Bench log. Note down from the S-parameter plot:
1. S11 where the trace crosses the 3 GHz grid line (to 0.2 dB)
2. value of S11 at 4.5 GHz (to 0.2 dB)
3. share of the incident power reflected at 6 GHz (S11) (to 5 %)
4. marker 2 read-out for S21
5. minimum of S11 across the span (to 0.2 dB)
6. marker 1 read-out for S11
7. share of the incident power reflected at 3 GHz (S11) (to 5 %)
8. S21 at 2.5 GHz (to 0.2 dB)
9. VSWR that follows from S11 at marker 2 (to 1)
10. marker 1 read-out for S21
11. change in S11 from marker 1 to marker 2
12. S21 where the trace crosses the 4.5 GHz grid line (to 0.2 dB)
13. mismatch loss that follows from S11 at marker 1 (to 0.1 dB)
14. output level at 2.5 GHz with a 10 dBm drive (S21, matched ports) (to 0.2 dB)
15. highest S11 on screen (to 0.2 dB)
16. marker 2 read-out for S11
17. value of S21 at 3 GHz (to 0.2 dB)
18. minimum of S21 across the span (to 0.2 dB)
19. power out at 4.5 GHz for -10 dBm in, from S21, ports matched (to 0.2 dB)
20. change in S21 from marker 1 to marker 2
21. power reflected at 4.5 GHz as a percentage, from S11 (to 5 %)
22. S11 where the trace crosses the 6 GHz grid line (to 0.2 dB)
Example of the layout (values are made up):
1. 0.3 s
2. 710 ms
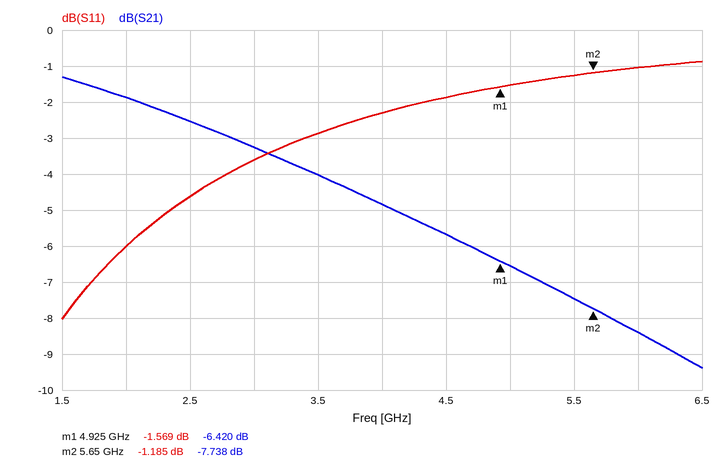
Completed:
1. -3.6 dB
2. -1.8 dB
3. 80 %
4. -7.738 dB
5. -8.0 dB
6. -1.569 dB
7. 45 %
8. -2.6 dB
9. 15
10. -6.420 dB
11. 0.384 dB
12. -5.6 dB
13. 5.2 dB
14. 7.4 dBm
15. -0.8 dB
16. -1.185 dB
17. -3.2 dB
18. -9.4 dB
19. -15.6 dBm
20. -1.318 dB
21. 65 %
22. -1.0 dB
